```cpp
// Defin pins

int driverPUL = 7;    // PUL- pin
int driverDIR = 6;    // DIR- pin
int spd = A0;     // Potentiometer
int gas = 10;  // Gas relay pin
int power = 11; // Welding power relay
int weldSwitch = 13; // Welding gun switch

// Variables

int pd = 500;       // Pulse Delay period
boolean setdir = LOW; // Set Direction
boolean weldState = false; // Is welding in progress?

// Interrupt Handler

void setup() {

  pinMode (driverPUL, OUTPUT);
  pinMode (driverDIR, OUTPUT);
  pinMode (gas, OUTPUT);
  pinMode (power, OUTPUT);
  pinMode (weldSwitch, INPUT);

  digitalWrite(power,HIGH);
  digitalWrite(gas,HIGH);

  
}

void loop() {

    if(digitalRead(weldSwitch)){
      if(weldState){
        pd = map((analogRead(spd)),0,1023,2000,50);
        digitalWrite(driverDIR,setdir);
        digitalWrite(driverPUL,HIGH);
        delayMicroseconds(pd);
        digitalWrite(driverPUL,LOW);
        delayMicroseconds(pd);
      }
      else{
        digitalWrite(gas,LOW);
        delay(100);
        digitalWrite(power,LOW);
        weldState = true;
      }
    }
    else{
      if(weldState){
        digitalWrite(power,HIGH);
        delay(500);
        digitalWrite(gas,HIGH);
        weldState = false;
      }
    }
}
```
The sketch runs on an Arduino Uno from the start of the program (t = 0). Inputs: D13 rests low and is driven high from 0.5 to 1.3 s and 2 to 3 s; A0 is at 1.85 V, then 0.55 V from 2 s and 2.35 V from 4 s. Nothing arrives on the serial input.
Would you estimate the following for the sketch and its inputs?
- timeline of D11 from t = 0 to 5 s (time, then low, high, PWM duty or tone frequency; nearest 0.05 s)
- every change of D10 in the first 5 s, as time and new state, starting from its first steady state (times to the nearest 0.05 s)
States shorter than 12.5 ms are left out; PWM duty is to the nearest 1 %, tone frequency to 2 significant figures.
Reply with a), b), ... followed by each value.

a) 0 s high; 0.6 s low; 1.3 s high; 2.1 s low; 3 s high
b) 0 s high; 0.5 s low; 1.8 s high; 2 s low; 3.5 s high
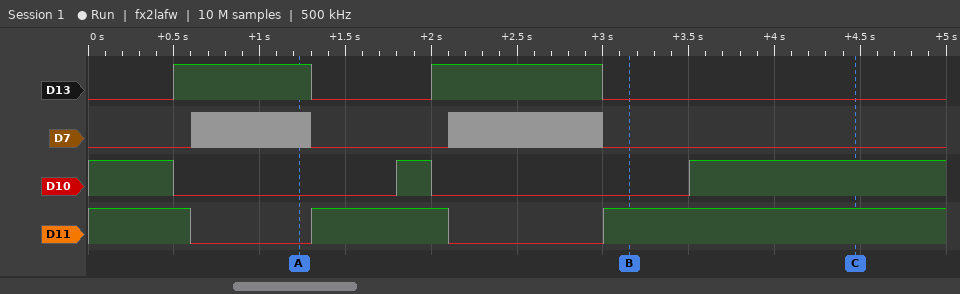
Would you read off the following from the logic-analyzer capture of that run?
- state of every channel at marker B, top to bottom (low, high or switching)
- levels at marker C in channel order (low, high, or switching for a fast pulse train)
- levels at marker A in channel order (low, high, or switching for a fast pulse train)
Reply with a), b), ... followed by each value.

a) D13 low, D7 low, D10 low, D11 high
b) D13 low, D7 low, D10 high, D11 high
c) D13 high, D7 switching, D10 low, D11 low
